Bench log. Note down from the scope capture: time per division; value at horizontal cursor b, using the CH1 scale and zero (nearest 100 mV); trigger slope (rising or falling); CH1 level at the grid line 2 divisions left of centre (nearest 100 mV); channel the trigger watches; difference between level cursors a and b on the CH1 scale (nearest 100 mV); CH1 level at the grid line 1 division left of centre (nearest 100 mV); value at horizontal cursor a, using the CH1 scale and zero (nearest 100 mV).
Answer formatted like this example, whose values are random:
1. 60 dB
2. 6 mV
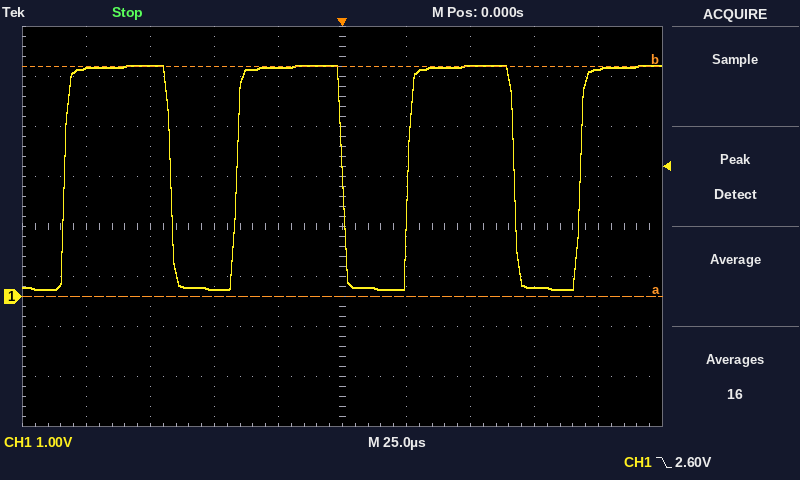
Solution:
1. 25 µs
2. 4.6 V
3. falling
4. 100 mV
5. CH1
6. 4.6 V
7. 4.6 V
8. 0.0 V
